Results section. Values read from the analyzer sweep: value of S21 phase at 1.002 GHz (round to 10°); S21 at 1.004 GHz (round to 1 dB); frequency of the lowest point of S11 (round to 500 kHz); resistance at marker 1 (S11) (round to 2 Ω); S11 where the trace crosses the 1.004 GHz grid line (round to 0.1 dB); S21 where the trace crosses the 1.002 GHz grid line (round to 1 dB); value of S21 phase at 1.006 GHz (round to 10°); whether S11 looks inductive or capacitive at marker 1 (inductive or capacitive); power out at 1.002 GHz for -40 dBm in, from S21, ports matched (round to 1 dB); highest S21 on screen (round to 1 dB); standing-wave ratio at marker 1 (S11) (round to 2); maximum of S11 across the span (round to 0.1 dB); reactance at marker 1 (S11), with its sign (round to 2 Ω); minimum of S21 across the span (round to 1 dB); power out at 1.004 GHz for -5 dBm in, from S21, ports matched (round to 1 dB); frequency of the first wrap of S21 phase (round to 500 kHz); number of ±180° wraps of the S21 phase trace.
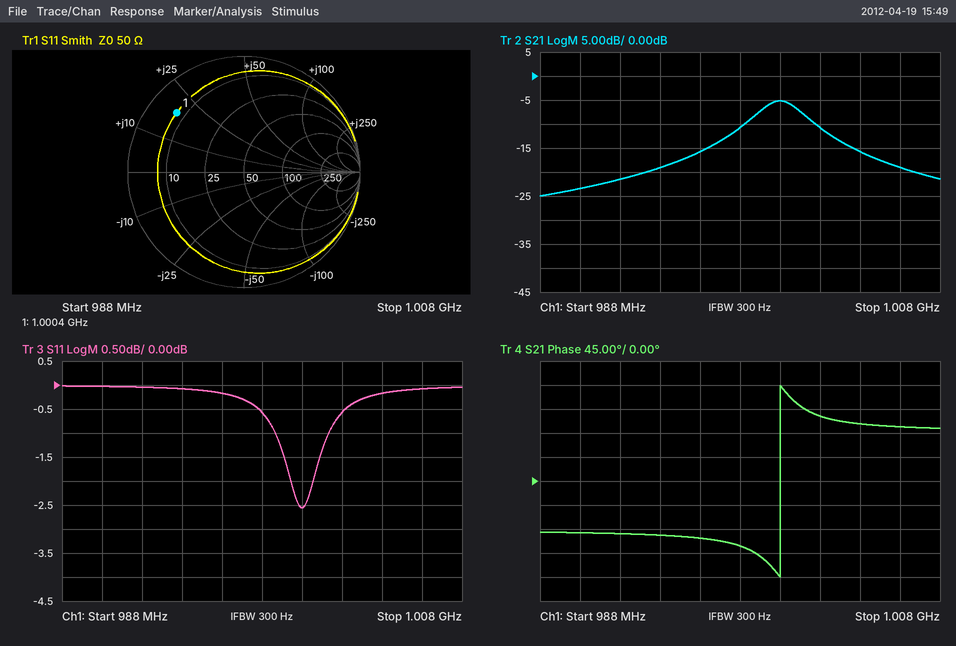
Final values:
120°
-16 dB
1.0000 GHz
8 Ω
-0.2 dB
-11 dB
100°
inductive
-51 dBm
-5 dB
8
0.0 dB
+18 Ω
-25 dB
-21 dBm
1.0000 GHz
1
